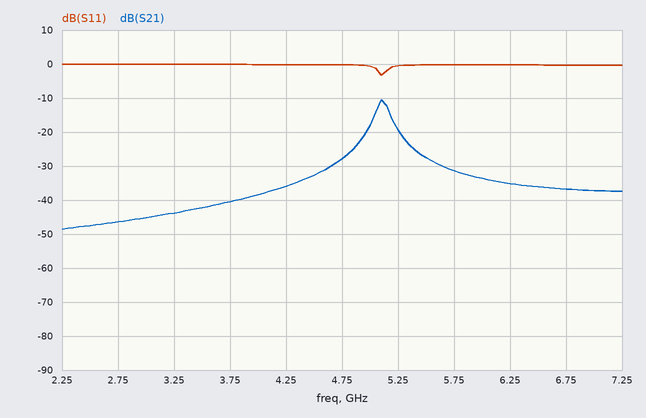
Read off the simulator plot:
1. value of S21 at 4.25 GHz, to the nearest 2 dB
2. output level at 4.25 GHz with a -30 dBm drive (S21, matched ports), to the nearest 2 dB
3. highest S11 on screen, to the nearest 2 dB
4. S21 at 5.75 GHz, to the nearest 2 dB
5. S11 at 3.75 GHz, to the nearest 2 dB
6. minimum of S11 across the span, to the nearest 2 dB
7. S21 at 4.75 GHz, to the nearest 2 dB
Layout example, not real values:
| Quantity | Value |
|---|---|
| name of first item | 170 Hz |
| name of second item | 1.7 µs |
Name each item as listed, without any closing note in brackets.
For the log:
| Quantity | Value |
|---|---|
| value of S21 at 4.25 GHz, to the nearest 2 dB | -36 dB |
| output level at 4.25 GHz with a -30 dBm drive (S21, matched ports), to the nearest 2 dB | -66 dBm |
| highest S11 on screen, to the nearest 2 dB | 0 dB |
| S21 at 5.75 GHz, to the nearest 2 dB | -32 dB |
| S11 at 3.75 GHz, to the nearest 2 dB | 0 dB |
| minimum of S11 across the span, to the nearest 2 dB | -4 dB |
| S21 at 4.75 GHz, to the nearest 2 dB | -28 dB |
